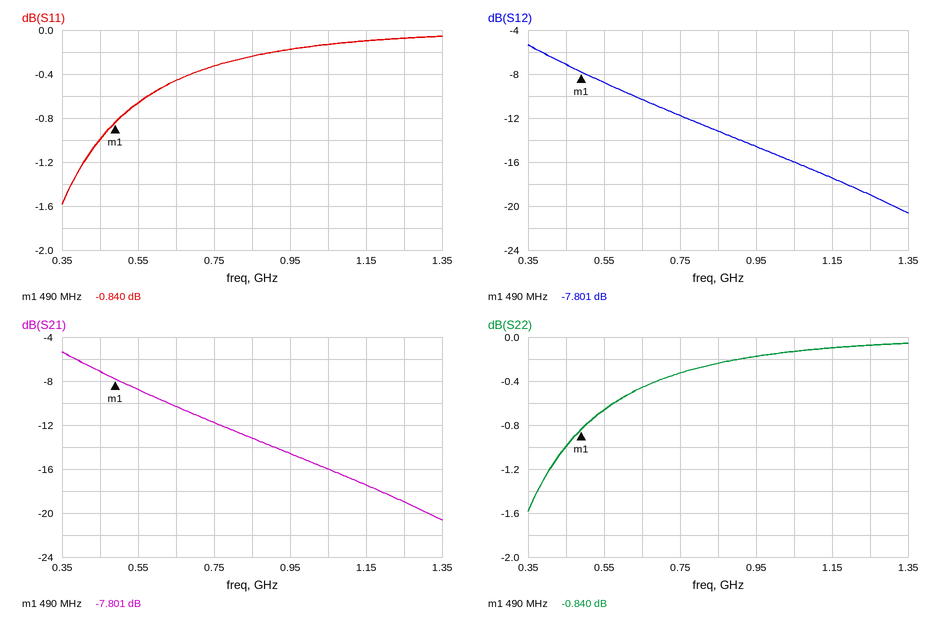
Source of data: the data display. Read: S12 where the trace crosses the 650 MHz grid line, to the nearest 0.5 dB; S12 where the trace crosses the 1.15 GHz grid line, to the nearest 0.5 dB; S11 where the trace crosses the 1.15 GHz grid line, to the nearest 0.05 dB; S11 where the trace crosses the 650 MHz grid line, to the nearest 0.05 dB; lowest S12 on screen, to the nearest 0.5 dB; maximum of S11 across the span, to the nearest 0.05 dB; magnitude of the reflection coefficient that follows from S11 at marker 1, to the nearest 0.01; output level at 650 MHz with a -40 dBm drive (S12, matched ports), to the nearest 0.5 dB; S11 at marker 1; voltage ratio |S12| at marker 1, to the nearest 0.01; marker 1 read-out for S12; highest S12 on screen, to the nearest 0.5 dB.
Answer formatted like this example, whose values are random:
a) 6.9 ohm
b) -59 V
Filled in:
a) -10.5 dB
b) -17.5 dB
c) -0.10 dB
d) -0.45 dB
e) -20.5 dB
f) -0.05 dB
g) 0.91
h) -50.5 dBm
i) -0.840 dB
j) 0.41
k) -7.801 dB
l) -5.5 dB
